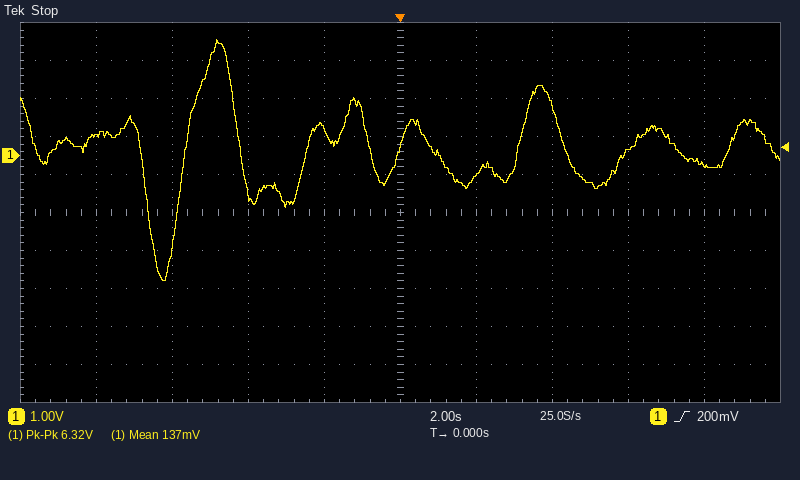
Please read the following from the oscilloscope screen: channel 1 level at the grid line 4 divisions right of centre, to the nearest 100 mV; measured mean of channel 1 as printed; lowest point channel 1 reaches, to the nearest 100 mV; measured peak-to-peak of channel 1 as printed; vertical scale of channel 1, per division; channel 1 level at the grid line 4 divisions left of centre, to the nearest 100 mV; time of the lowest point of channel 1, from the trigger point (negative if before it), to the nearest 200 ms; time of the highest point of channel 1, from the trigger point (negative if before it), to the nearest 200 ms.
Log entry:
-200 mV
137 mV
-3.3 V
6.32 V
1 V
600 mV
-6.2 s
-4.8 s
